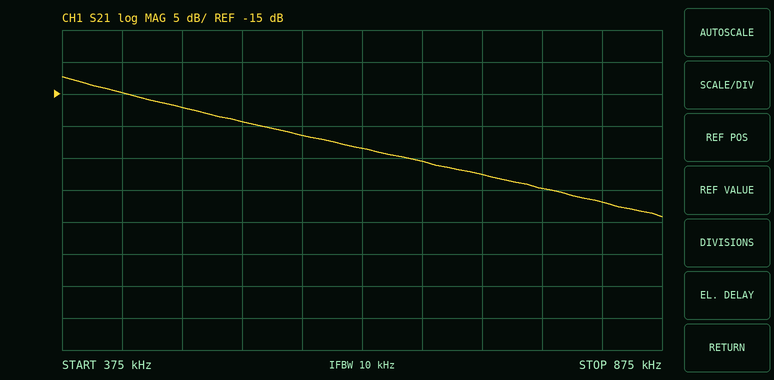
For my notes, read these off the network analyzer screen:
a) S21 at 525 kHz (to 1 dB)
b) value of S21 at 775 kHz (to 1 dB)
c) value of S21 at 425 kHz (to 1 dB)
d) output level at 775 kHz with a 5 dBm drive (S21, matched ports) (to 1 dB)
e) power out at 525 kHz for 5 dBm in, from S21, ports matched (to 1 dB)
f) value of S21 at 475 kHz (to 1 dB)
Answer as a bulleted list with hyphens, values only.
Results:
- -19 dB
- -30 dB
- -15 dB
- -25 dBm
- -14 dBm
- -17 dB
